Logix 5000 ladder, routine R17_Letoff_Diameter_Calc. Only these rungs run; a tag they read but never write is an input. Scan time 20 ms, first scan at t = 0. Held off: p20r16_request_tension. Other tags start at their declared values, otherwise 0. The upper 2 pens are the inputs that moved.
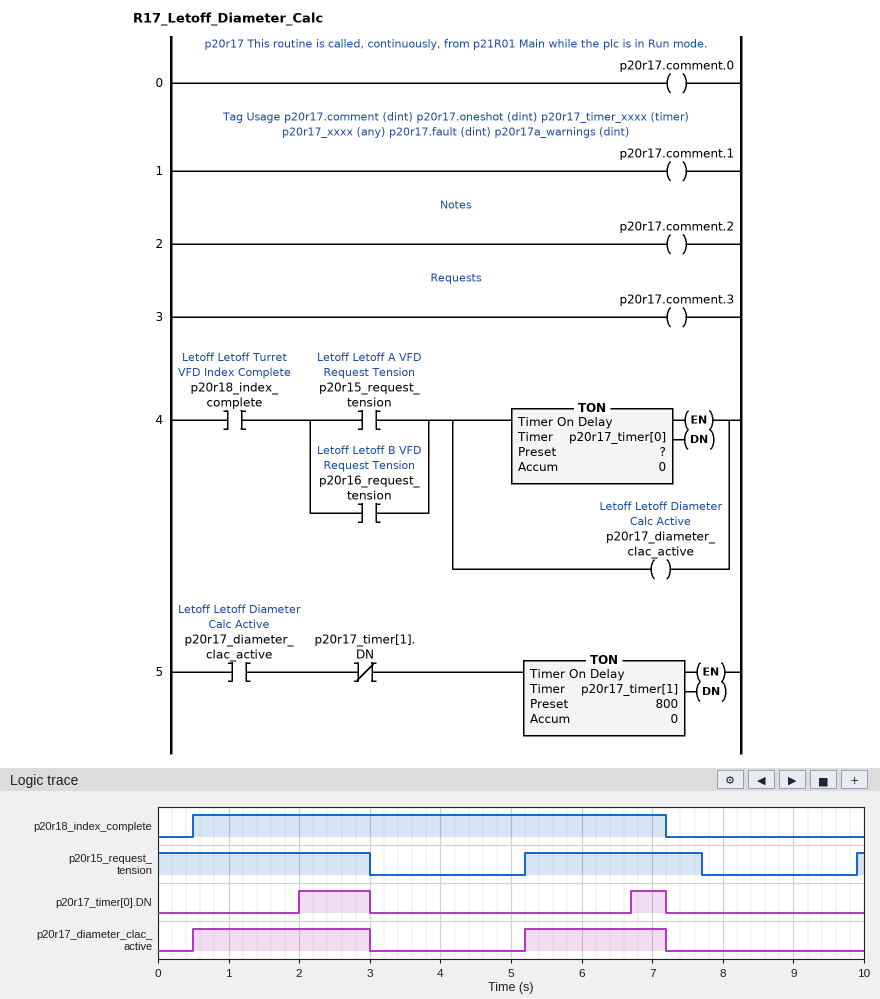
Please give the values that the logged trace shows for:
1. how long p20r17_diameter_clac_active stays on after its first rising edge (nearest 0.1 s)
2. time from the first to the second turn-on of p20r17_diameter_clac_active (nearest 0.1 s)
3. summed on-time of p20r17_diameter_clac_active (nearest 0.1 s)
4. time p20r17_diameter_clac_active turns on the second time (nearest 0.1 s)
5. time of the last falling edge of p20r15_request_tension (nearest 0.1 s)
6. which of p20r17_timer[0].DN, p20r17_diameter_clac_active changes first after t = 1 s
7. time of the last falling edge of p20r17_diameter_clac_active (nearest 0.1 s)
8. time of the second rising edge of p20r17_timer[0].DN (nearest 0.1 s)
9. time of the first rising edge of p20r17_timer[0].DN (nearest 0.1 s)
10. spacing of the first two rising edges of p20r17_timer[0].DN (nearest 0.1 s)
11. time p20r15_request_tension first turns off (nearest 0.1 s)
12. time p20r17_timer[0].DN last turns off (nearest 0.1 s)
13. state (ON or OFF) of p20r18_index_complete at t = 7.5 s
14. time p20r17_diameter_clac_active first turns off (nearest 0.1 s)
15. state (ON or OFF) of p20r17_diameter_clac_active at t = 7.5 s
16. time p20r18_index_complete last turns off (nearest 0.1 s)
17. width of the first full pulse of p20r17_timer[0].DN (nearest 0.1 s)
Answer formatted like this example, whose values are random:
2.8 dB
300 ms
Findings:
2.5 s
4.7 s
4.5 s
5.2 s
7.7 s
p20r17_timer[0].DN
7.2 s
6.7 s
2.0 s
4.7 s
3.0 s
7.2 s
OFF
3.0 s
OFF
7.2 s
1.0 s
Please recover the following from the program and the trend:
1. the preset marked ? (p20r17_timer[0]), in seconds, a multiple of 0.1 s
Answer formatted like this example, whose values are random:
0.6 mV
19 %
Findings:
1.5 s
